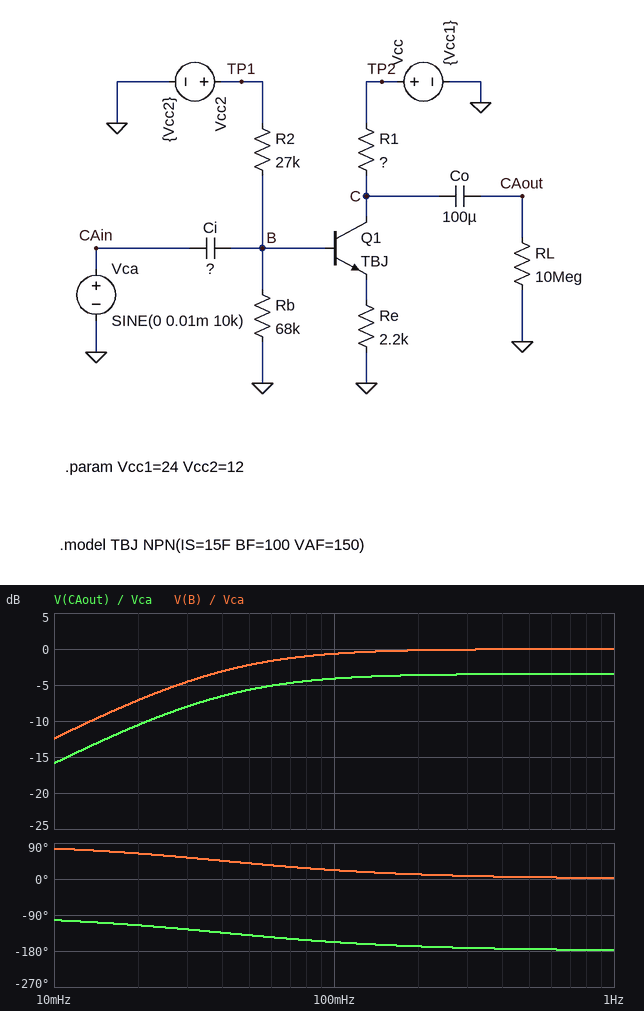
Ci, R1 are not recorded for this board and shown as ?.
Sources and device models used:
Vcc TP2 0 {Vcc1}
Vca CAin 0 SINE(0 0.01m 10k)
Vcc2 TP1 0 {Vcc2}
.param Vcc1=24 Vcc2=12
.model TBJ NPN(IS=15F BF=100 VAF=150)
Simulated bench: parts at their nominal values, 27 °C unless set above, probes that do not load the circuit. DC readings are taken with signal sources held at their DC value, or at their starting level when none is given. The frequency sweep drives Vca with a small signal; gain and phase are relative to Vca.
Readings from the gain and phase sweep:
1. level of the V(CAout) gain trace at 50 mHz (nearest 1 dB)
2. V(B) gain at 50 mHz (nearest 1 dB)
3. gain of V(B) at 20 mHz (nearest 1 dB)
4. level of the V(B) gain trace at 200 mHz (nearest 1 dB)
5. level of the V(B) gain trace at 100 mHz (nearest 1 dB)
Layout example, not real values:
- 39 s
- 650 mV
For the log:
- -6 dB
- -2 dB
- -7 dB
- 0 dB
- -1 dB
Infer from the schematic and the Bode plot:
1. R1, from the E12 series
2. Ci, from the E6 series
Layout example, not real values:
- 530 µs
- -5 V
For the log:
- 1.5 kΩ
- 220 µF
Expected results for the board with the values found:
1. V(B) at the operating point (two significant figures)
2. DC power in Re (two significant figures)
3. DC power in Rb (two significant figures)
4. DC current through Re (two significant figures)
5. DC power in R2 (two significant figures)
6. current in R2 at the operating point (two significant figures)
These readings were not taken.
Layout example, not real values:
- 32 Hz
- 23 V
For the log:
- 8.0 V
- 24 mW
- 940 µW
- 3.3 mA
- 590 µW
- 150 µA
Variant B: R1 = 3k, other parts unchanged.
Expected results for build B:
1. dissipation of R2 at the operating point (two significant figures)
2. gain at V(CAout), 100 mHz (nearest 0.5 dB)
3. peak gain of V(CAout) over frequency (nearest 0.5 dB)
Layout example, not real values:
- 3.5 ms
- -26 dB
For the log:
- 600 µW
- 2.0 dB
- 2.5 dB
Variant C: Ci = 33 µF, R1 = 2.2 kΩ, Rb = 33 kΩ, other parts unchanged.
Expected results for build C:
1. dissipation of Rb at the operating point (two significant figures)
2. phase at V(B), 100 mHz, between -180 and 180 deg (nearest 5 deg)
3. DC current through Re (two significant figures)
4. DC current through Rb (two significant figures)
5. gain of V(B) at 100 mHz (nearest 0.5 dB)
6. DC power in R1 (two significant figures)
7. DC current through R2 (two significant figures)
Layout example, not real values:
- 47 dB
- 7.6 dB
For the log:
- 1.2 mW
- 75 deg
- 2.5 mA
- 190 µA
- -11.0 dB
- 14 mW
- 210 µA
